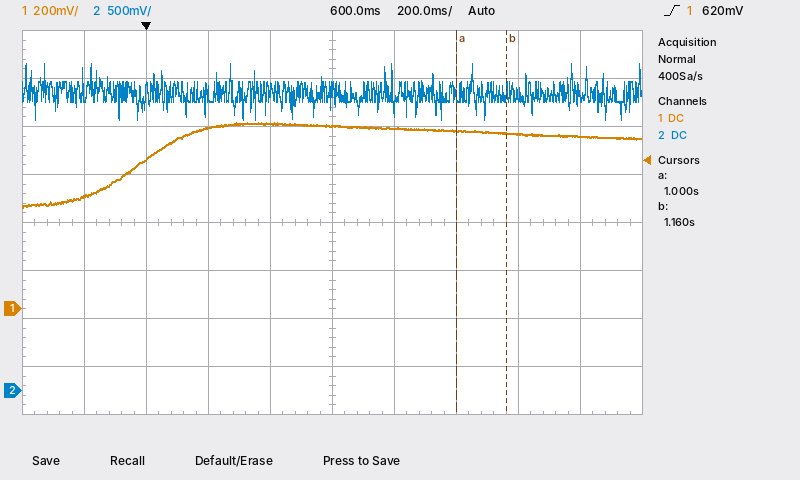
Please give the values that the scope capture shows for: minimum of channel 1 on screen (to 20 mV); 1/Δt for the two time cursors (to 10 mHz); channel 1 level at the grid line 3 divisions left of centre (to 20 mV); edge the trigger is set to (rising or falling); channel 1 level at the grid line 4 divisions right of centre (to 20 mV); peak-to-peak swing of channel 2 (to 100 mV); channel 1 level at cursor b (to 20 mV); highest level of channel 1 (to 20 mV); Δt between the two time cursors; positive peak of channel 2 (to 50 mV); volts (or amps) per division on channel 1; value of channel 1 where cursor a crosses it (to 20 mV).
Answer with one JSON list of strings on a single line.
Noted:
["420 mV", "6.25 Hz", "620 mV", "rising", "720 mV", "600 mV", "740 mV", "780 mV", "160 ms", "3.40 V", "200 mV", "740 mV"]
